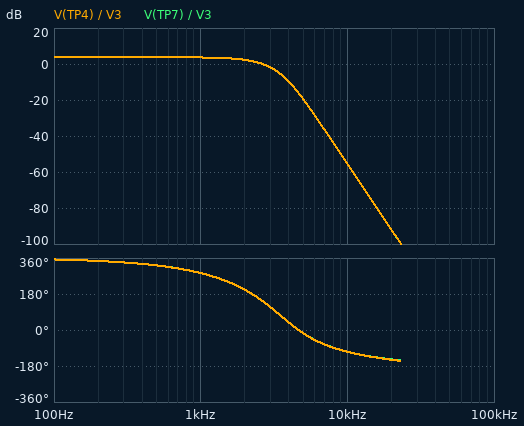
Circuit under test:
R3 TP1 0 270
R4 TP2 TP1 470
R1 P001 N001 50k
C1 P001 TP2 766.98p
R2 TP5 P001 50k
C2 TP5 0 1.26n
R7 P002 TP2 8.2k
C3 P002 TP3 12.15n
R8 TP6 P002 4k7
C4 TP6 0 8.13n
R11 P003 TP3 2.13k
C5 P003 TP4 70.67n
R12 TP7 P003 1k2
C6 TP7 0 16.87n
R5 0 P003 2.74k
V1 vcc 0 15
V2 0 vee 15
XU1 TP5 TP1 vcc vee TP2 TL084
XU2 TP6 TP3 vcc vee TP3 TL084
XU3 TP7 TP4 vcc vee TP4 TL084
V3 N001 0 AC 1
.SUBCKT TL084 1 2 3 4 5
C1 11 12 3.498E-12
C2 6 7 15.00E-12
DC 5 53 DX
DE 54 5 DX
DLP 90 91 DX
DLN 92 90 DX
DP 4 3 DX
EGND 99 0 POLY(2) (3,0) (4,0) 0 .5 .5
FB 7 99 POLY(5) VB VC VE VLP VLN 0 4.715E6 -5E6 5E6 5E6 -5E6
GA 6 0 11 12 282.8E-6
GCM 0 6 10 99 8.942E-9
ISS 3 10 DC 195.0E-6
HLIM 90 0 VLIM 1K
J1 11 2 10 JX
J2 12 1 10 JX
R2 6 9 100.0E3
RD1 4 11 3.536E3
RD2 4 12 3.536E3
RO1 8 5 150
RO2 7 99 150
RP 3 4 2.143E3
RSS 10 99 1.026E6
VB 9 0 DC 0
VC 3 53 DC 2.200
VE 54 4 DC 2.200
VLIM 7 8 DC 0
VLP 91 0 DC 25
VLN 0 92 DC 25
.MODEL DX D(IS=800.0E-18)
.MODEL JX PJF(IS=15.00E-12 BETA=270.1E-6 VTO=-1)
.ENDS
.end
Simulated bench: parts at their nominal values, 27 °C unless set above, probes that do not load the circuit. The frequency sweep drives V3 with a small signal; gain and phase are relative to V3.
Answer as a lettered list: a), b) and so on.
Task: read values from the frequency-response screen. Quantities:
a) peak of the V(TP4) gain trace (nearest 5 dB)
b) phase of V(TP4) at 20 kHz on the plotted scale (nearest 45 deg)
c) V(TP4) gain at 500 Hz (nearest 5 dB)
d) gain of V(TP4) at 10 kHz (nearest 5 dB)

a) 5 dB
b) -135 deg
c) 5 dB
d) -55 dB
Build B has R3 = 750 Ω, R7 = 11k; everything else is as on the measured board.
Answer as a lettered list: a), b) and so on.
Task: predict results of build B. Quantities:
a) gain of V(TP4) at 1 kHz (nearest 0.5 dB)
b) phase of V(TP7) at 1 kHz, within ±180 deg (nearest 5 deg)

a) -2.5 dB
b) -95 deg
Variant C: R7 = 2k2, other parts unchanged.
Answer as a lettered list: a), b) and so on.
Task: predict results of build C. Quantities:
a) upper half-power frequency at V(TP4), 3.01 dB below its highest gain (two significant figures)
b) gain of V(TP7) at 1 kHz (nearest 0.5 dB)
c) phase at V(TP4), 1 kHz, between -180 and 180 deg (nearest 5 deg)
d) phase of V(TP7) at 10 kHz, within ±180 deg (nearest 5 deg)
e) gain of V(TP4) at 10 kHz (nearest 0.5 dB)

a) 3.2 kHz
b) 4.0 dB
c) -60 deg
d) -85 deg
e) -45.0 dB
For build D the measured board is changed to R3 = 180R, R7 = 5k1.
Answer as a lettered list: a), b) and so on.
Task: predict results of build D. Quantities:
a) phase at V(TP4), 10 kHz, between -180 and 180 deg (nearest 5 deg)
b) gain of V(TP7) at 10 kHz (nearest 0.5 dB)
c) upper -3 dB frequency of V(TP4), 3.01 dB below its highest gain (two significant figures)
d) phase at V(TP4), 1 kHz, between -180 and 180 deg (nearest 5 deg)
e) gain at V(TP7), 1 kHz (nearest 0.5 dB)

a) -115 deg
b) -48.5 dB
c) 3.4 kHz
d) -55 deg
e) 7.0 dB
